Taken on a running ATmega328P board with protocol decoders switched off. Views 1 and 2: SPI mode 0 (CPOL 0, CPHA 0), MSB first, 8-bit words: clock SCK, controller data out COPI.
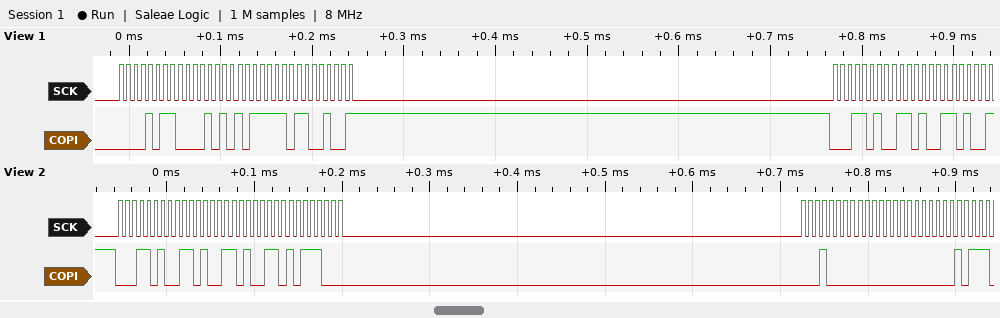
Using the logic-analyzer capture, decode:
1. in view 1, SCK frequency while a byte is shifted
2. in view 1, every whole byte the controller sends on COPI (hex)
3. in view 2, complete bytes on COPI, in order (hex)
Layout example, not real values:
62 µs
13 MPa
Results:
125 kHz
0x0B 0x0A 0xBE 0xC9 0x1A 0x69
0x1A 0x69 0xA6 0xB8 0x10 0x00 0x02
